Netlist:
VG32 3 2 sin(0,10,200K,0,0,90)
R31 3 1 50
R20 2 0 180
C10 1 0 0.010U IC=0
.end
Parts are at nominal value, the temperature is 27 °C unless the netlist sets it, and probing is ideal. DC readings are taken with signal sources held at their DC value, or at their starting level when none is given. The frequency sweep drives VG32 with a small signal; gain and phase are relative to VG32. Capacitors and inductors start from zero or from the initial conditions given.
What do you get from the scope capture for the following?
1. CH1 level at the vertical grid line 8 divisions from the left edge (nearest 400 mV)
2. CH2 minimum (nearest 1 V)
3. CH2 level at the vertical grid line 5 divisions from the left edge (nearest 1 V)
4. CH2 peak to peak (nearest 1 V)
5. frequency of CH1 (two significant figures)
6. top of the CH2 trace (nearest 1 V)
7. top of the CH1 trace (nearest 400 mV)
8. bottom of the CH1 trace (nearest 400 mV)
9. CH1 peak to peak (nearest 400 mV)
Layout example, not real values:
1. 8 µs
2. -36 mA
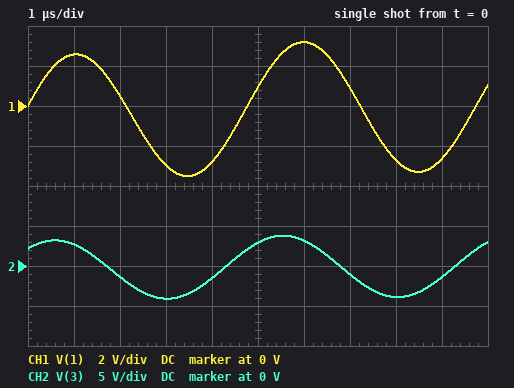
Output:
1. -2.8 V
2. -4 V
3. 3 V
4. 8 V
5. 200 kHz
6. 4 V
7. 3.2 V
8. -3.6 V
9. 6.8 V
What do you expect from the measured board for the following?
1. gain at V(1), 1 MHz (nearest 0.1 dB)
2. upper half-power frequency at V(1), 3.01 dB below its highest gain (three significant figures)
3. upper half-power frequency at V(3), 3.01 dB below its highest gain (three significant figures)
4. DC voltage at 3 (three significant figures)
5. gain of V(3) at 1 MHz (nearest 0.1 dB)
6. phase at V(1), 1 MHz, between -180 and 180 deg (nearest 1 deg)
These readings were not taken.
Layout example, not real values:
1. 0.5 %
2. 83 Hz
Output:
1. -23.2 dB
2. 69.2 kHz
3. 72.7 kHz
4. 10.0 V
5. -12.9 dB
6. -86 deg
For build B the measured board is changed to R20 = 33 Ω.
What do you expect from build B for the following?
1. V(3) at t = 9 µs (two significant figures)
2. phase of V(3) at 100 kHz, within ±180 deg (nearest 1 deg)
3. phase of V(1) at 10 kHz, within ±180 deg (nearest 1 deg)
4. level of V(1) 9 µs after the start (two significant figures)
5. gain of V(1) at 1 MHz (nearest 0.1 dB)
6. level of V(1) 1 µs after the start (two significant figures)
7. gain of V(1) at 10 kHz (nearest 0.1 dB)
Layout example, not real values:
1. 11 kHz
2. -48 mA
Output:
1. 560 mV
2. -10 deg
3. -3 deg
4. -3.3 V
5. -14.5 dB
6. 4.8 V
7. 0 dB
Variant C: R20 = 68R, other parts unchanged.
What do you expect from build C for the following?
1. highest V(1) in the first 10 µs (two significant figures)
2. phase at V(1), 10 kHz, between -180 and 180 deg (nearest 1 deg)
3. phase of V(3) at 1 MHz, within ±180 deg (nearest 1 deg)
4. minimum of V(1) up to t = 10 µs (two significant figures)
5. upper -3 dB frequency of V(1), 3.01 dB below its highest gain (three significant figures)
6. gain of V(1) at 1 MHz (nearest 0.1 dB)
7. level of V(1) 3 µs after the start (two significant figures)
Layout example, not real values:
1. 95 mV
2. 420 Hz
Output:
1. 5.6 V
2. -4 deg
3. -10 deg
4. -5.8 V
5. 135 kHz
6. -17.5 dB
7. -5.5 V
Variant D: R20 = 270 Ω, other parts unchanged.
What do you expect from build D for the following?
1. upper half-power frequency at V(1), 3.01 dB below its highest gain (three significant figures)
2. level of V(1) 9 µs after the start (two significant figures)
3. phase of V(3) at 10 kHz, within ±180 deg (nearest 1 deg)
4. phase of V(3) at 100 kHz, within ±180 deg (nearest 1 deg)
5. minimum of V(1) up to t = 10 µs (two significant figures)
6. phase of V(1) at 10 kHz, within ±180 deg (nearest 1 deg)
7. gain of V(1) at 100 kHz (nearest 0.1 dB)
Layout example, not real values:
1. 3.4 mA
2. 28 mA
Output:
1. 49.7 kHz
2. -2.1 V
3. -10 deg
4. -46 deg
5. -2.6 V
6. -11 deg
7. -7.0 dB
